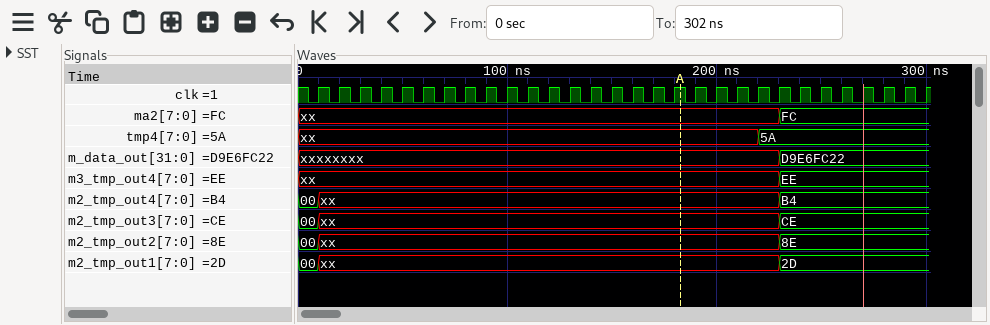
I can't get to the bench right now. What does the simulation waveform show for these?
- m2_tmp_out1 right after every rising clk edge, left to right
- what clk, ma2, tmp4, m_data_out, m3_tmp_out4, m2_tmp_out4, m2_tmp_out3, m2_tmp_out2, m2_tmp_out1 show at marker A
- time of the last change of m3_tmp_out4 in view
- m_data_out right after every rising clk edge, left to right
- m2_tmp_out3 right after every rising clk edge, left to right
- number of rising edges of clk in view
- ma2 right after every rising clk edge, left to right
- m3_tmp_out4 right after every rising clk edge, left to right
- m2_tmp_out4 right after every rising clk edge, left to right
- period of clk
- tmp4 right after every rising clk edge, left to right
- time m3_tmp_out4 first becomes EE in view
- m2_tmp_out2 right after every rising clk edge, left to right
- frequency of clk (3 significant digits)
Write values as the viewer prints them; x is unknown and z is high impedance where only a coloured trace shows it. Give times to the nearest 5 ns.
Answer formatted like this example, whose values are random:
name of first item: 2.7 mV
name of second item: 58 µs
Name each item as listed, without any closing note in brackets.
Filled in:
m2_tmp_out1 right after every rising clk edge, left to right: xx, xx, xx, xx, xx, xx, xx, xx, xx, xx, xx, xx, xx, xx, xx, xx, xx, xx, xx, xx, xx, xx, 2D, 2D, 2D, 2D, 2D, 2D, 2D, 2D
what clk, ma2, tmp4, m_data_out, m3_tmp_out4, m2_tmp_out4, m2_tmp_out3, m2_tmp_out2, m2_tmp_out1 show at marker A: clk=1, ma2=xx, tmp4=xx, m_data_out=xxxxxxxx, m3_tmp_out4=xx, m2_tmp_out4=xx, m2_tmp_out3=xx, m2_tmp_out2=xx, m2_tmp_out1=xx
time of the last change of m3_tmp_out4 in view: 230 ns
m_data_out right after every rising clk edge, left to right: xxxxxxxx, xxxxxxxx, xxxxxxxx, xxxxxxxx, xxxxxxxx, xxxxxxxx, xxxxxxxx, xxxxxxxx, xxxxxxxx, xxxxxxxx, xxxxxxxx, xxxxxxxx, xxxxxxxx, xxxxxxxx, xxxxxxxx, xxxxxxxx, xxxxxxxx, xxxxxxxx, xxxxxxxx, xxxxxxxx, xxxxxxxx, xxxxxxxx, D9E6FC22, D9E6FC22, D9E6FC22, D9E6FC22, D9E6FC22, D9E6FC22, D9E6FC22, D9E6FC22
m2_tmp_out3 right after every rising clk edge, left to right: xx, xx, xx, xx, xx, xx, xx, xx, xx, xx, xx, xx, xx, xx, xx, xx, xx, xx, xx, xx, xx, xx, CE, CE, CE, CE, CE, CE, CE, CE
number of rising edges of clk in view: 30
ma2 right after every rising clk edge, left to right: xx, xx, xx, xx, xx, xx, xx, xx, xx, xx, xx, xx, xx, xx, xx, xx, xx, xx, xx, xx, xx, xx, FC, FC, FC, FC, FC, FC, FC, FC
m3_tmp_out4 right after every rising clk edge, left to right: xx, xx, xx, xx, xx, xx, xx, xx, xx, xx, xx, xx, xx, xx, xx, xx, xx, xx, xx, xx, xx, xx, EE, EE, EE, EE, EE, EE, EE, EE
m2_tmp_out4 right after every rising clk edge, left to right: xx, xx, xx, xx, xx, xx, xx, xx, xx, xx, xx, xx, xx, xx, xx, xx, xx, xx, xx, xx, xx, xx, B4, B4, B4, B4, B4, B4, B4, B4
period of clk: 10 ns
tmp4 right after every rising clk edge, left to right: xx, xx, xx, xx, xx, xx, xx, xx, xx, xx, xx, xx, xx, xx, xx, xx, xx, xx, xx, xx, xx, 5A, 5A, 5A, 5A, 5A, 5A, 5A, 5A, 5A
time m3_tmp_out4 first becomes EE in view: 230 ns
m2_tmp_out2 right after every rising clk edge, left to right: xx, xx, xx, xx, xx, xx, xx, xx, xx, xx, xx, xx, xx, xx, xx, xx, xx, xx, xx, xx, xx, xx, 8E, 8E, 8E, 8E, 8E, 8E, 8E, 8E
frequency of clk: 100 MHz
